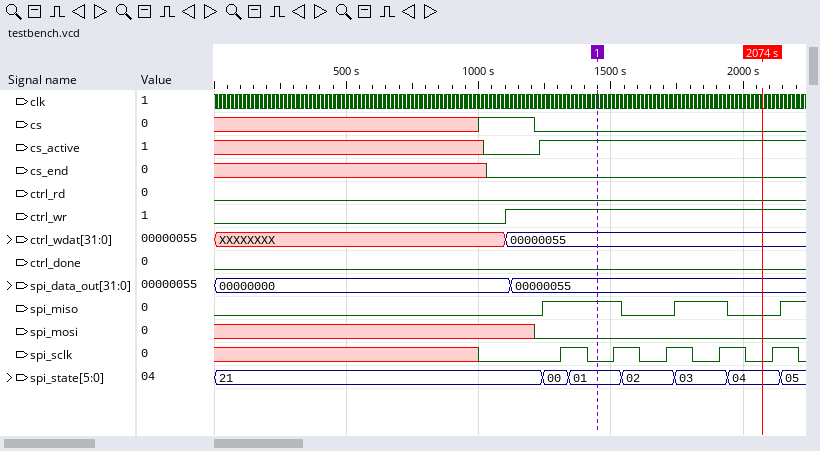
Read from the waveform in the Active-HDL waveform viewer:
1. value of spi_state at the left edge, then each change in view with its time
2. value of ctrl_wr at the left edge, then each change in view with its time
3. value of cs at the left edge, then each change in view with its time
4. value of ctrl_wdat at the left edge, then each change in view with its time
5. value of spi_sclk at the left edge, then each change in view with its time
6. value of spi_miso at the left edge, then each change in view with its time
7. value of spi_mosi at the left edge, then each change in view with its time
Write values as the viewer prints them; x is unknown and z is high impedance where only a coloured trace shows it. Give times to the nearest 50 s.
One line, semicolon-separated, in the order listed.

21, 00 at 1250 s, 01 at 1350 s, 02 at 1550 s, 03 at 1750 s, 04 at 1950 s, 05 at 2150 s; 0, 1 at 1100 s; x, 1 at 1000 s, 0 at 1200 s; XXXXXXXX, 00000055 at 1100 s; x, 0 at 1000 s, 1 at 1300 s, 0 at 1400 s, 1 at 1500 s, 0 at 1600 s, 1 at 1700 s, 0 at 1800 s, 1 at 1900 s, 0 at 2000 s, 1 at 2100 s, 0 at 2200 s; 0, 1 at 1250 s, 0 at 1550 s, 1 at 1750 s, 0 at 1950 s, 1 at 2150 s; x, 0 at 1200 s
